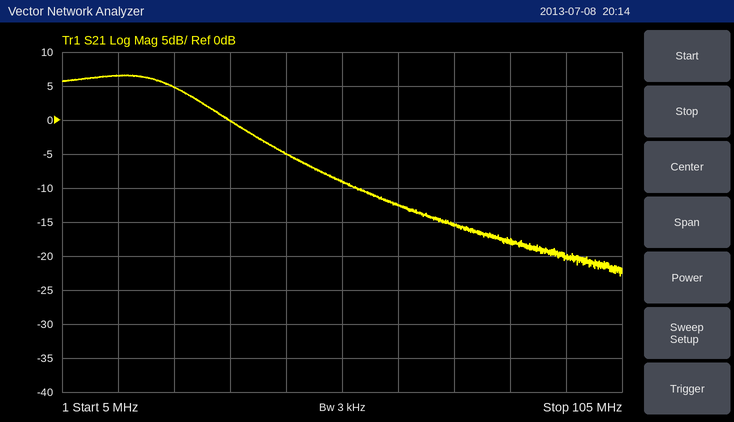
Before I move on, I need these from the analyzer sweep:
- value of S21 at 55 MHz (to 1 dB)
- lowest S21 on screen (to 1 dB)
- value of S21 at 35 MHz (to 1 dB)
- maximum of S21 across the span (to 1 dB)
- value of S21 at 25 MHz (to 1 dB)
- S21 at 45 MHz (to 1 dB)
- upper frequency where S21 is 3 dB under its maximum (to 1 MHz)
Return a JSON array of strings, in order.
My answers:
["-9 dB", "-23 dB", "0 dB", "7 dB", "5 dB", "-5 dB", "28 MHz"]
